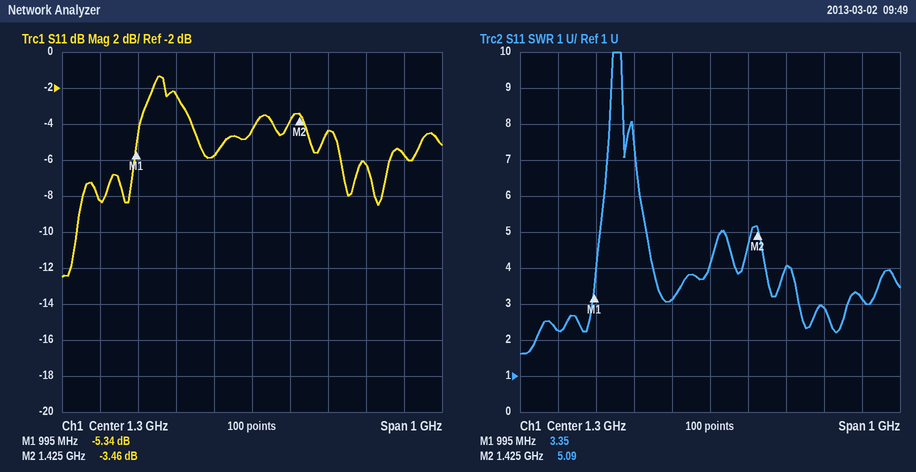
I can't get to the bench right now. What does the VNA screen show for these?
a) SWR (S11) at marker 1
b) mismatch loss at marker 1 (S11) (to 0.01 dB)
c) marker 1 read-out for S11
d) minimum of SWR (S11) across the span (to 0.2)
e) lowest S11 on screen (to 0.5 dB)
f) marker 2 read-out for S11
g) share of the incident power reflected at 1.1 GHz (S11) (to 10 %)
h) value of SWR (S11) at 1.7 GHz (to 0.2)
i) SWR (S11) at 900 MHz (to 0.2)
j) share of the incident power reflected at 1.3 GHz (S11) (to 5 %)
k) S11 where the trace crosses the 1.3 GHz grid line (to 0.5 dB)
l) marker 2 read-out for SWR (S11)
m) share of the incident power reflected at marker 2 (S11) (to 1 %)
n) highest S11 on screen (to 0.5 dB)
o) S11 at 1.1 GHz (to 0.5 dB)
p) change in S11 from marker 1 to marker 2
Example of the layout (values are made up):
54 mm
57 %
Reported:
3.35
1.50 dB
-5.34 dB
1.6
-12.5 dB
-3.46 dB
60 %
3.2
2.2
35 %
-4.5 dB
5.09
45 %
-1.5 dB
-2.5 dB
1.88 dB
